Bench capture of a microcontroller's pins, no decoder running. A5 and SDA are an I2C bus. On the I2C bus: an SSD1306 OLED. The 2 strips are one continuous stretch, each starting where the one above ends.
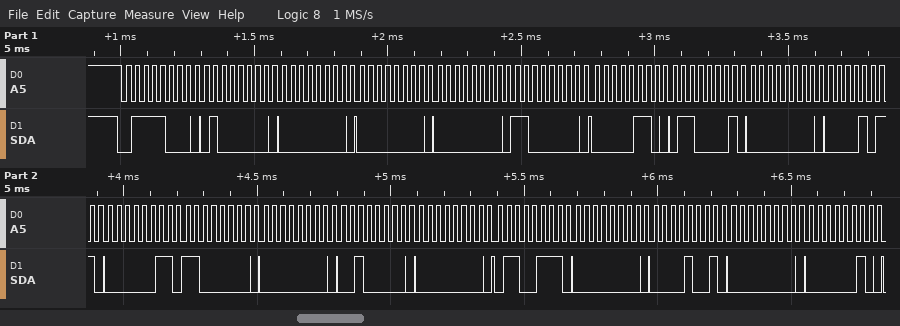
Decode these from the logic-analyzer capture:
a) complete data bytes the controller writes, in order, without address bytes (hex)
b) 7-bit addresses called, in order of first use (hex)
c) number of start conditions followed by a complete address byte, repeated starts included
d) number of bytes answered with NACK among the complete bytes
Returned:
40 00 00 00 C0 06 61 00 0B 03 C0 00 20 00 67 00 09 00 02
0x3C
1
0
